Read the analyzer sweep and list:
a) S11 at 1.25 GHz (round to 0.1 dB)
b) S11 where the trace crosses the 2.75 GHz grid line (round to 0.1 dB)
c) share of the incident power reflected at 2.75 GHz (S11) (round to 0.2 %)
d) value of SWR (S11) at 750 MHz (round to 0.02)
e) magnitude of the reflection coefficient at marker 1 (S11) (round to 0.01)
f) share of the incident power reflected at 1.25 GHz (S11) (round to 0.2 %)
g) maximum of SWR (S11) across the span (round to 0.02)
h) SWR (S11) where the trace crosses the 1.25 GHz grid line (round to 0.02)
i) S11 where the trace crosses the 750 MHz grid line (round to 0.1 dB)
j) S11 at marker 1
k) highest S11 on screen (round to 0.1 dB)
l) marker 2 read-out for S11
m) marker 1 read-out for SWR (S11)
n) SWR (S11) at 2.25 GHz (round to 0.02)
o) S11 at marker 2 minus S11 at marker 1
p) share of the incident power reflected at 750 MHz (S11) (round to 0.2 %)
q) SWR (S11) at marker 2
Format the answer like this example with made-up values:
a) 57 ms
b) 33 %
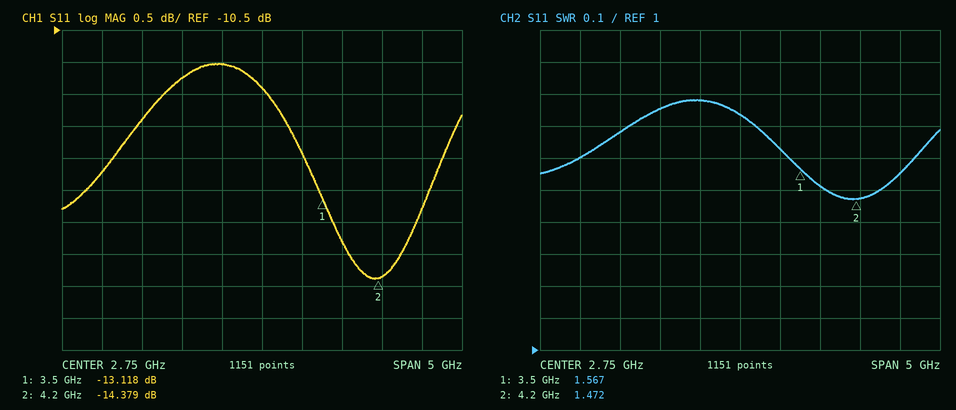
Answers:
a) -11.9 dB
b) -11.4 dB
c) 7.2 %
d) 1.60
e) 0.22
f) 6.4 %
g) 1.78
h) 1.68
i) -12.7 dB
j) -13.118 dB
k) -11.0 dB
l) -14.379 dB
m) 1.567
n) 1.78
o) -1.261 dB
p) 5.4 %
q) 1.472
